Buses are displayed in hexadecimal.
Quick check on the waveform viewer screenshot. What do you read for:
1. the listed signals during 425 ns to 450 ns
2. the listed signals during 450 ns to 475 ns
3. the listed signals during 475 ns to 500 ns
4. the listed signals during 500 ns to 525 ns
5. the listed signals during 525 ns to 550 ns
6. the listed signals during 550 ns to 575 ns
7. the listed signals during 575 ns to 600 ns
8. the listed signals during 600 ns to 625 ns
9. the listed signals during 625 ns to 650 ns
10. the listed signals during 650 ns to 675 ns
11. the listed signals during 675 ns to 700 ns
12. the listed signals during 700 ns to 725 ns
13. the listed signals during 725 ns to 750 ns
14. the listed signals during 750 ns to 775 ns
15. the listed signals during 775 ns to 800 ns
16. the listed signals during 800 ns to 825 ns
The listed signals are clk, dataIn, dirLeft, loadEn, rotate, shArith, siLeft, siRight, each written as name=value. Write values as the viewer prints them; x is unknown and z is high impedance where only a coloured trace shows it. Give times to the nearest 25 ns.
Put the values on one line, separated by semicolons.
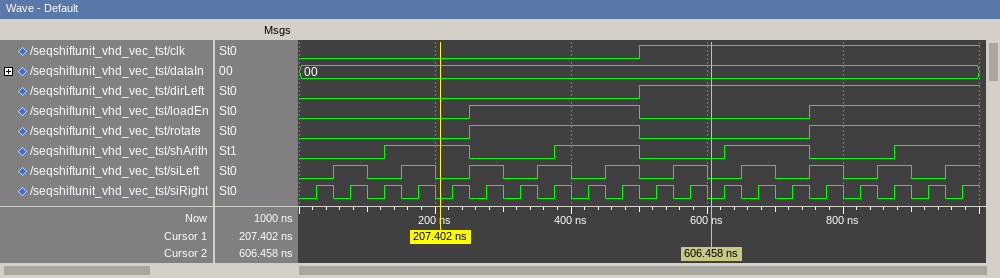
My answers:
clk=0, dataIn=00, dirLeft=0, loadEn=1, rotate=1, shArith=1, siLeft=0, siRight=1; clk=0, dataIn=00, dirLeft=0, loadEn=1, rotate=1, shArith=1, siLeft=1, siRight=0; clk=0, dataIn=00, dirLeft=0, loadEn=1, rotate=1, shArith=1, siLeft=1, siRight=1; clk=1, dataIn=00, dirLeft=1, loadEn=0, rotate=0, shArith=0, siLeft=0, siRight=0; clk=1, dataIn=00, dirLeft=1, loadEn=0, rotate=0, shArith=0, siLeft=0, siRight=1; clk=1, dataIn=00, dirLeft=1, loadEn=0, rotate=0, shArith=0, siLeft=1, siRight=0; clk=1, dataIn=00, dirLeft=1, loadEn=0, rotate=0, shArith=0, siLeft=1, siRight=1; clk=1, dataIn=00, dirLeft=1, loadEn=0, rotate=0, shArith=0, siLeft=0, siRight=0; clk=1, dataIn=00, dirLeft=1, loadEn=0, rotate=0, shArith=1, siLeft=0, siRight=1; clk=1, dataIn=00, dirLeft=1, loadEn=0, rotate=0, shArith=1, siLeft=1, siRight=0; clk=1, dataIn=00, dirLeft=1, loadEn=0, rotate=0, shArith=1, siLeft=1, siRight=1; clk=1, dataIn=00, dirLeft=1, loadEn=0, rotate=0, shArith=1, siLeft=0, siRight=0; clk=1, dataIn=00, dirLeft=1, loadEn=0, rotate=0, shArith=1, siLeft=0, siRight=1; clk=1, dataIn=00, dirLeft=1, loadEn=1, rotate=1, shArith=0, siLeft=1, siRight=0; clk=1, dataIn=00, dirLeft=1, loadEn=1, rotate=1, shArith=0, siLeft=1, siRight=1; clk=1, dataIn=00, dirLeft=1, loadEn=1, rotate=1, shArith=0, siLeft=0, siRight=0
